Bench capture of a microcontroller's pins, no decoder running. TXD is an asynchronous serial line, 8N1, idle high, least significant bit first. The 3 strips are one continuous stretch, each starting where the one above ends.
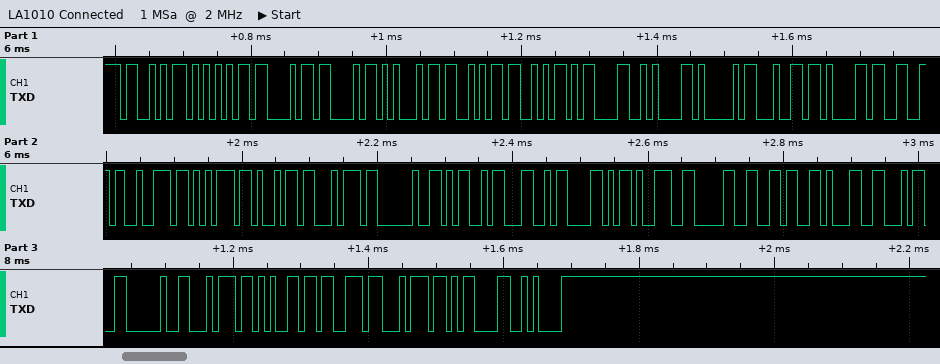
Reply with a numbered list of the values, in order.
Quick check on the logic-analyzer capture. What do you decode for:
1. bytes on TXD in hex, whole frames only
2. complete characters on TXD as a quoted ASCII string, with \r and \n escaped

1. 53 55 43 43 45 53 53 0D 0A 41 64 61 66 72 75 69 74 20 4D 4C 58 39 30 36 31 34 20 74 65 73 74 0D 0A
2. "SUCCESS\r\nAdafruit MLX90614 test\r\n"
